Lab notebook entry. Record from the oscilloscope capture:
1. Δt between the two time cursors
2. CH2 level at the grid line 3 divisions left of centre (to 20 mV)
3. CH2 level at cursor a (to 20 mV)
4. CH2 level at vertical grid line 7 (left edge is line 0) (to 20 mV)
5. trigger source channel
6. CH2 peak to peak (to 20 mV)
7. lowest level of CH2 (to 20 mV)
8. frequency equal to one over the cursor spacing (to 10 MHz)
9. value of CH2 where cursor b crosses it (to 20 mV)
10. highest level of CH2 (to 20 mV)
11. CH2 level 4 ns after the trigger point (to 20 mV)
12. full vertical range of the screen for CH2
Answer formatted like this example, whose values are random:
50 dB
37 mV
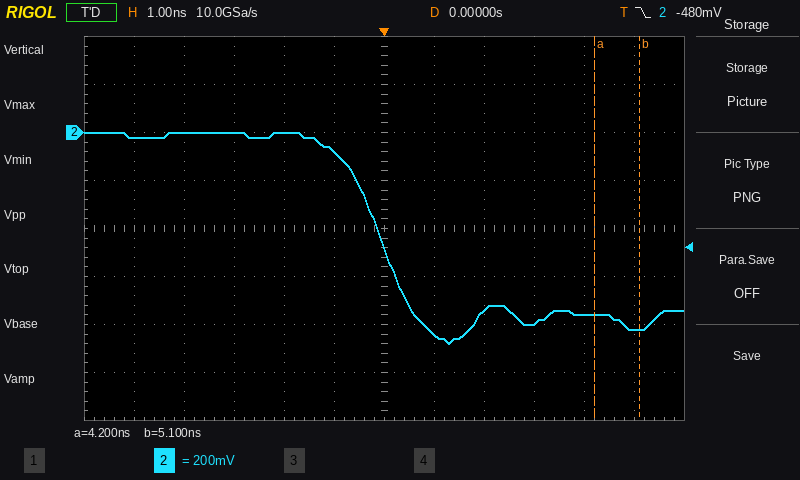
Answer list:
900 ps
0 mV
-760 mV
-840 mV
CH2
880 mV
-880 mV
1.11 GHz
-820 mV
0 mV
-760 mV
1.6 V
